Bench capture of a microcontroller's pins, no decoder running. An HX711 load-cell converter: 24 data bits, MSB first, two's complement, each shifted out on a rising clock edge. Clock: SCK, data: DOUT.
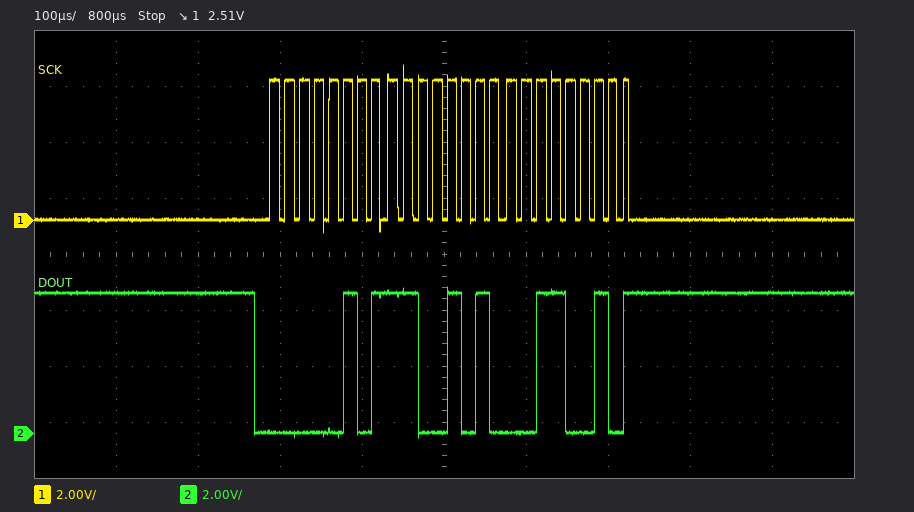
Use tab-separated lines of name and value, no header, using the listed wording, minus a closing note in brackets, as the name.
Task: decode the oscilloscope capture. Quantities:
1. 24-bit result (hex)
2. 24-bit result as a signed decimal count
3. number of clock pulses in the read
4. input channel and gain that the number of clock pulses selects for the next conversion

24-bit result	0x05CA32
24-bit result as a signed decimal count	379442
number of clock pulses in the read	25
input channel and gain that the number of clock pulses selects for the next conversion	channel A, gain 128
